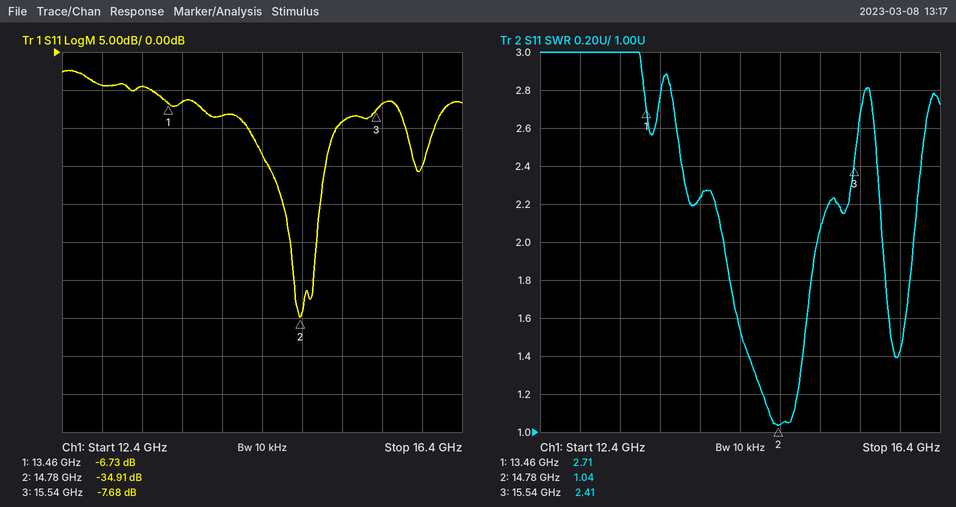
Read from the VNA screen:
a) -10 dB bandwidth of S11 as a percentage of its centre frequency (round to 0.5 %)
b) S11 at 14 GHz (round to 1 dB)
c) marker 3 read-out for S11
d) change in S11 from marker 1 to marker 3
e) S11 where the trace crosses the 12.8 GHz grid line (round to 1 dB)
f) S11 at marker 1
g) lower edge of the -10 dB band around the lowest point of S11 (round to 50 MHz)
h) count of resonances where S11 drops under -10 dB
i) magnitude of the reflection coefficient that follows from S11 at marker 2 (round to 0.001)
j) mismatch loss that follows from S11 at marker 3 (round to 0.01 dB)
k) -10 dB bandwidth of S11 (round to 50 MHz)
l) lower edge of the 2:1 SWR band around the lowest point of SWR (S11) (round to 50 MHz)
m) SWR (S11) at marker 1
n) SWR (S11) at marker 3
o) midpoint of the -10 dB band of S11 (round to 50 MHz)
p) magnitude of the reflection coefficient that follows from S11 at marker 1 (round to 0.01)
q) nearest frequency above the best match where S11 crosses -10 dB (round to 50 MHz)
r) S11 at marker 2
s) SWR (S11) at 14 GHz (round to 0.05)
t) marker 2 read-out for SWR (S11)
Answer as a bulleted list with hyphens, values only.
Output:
- 6.0 %
- -8 dB
- -7.68 dB
- -0.95 dB
- -4 dB
- -6.73 dB
- 14.25 GHz
- 2
- 0.018
- 0.81 dB
- 900 MHz
- 14.25 GHz
- 2.71
- 2.41
- 14.70 GHz
- 0.46
- 15.15 GHz
- -34.91 dB
- 2.25
- 1.04
